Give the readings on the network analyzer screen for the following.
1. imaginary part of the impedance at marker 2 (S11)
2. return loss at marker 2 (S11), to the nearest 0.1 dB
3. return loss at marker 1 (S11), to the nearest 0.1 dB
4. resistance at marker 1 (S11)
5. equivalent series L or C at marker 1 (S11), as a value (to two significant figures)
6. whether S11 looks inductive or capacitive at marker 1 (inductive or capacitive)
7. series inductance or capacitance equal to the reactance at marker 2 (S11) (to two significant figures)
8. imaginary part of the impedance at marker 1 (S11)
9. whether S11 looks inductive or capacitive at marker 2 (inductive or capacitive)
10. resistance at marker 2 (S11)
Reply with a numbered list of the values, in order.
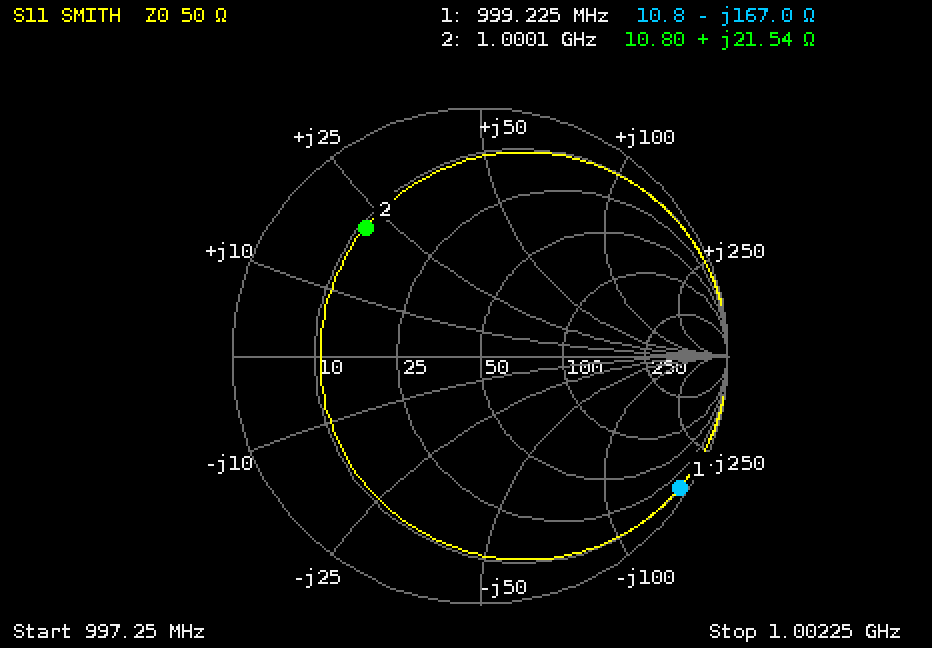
1. +21.54 Ω
2. 3.2 dB
3. 0.3 dB
4. 10.8 Ω
5. 950 fF
6. capacitive
7. 3.4 nH
8. -167.0 Ω
9. inductive
10. 10.80 Ω
